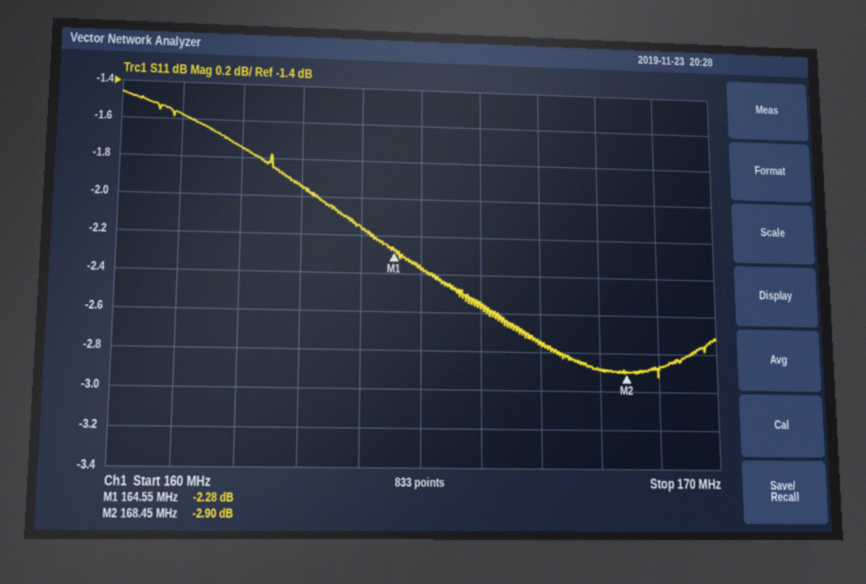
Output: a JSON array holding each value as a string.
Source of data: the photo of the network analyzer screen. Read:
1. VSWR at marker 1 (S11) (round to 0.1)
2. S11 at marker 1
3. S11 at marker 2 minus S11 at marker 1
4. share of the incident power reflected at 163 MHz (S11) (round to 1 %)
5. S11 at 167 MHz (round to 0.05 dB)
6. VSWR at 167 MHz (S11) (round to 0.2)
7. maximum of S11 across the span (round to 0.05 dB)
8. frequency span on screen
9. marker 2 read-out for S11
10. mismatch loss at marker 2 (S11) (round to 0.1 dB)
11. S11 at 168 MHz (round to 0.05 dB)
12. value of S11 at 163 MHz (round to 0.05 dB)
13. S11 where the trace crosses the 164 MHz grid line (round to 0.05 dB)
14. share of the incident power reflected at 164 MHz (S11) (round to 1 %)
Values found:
["7.7", "-2.28 dB", "-0.62 dB", "64 %", "-2.75 dB", "6.4", "-1.45 dB", "10 MHz", "-2.90 dB", "3.1 dB", "-2.90 dB", "-1.95 dB", "-2.15 dB", "61 %"]
